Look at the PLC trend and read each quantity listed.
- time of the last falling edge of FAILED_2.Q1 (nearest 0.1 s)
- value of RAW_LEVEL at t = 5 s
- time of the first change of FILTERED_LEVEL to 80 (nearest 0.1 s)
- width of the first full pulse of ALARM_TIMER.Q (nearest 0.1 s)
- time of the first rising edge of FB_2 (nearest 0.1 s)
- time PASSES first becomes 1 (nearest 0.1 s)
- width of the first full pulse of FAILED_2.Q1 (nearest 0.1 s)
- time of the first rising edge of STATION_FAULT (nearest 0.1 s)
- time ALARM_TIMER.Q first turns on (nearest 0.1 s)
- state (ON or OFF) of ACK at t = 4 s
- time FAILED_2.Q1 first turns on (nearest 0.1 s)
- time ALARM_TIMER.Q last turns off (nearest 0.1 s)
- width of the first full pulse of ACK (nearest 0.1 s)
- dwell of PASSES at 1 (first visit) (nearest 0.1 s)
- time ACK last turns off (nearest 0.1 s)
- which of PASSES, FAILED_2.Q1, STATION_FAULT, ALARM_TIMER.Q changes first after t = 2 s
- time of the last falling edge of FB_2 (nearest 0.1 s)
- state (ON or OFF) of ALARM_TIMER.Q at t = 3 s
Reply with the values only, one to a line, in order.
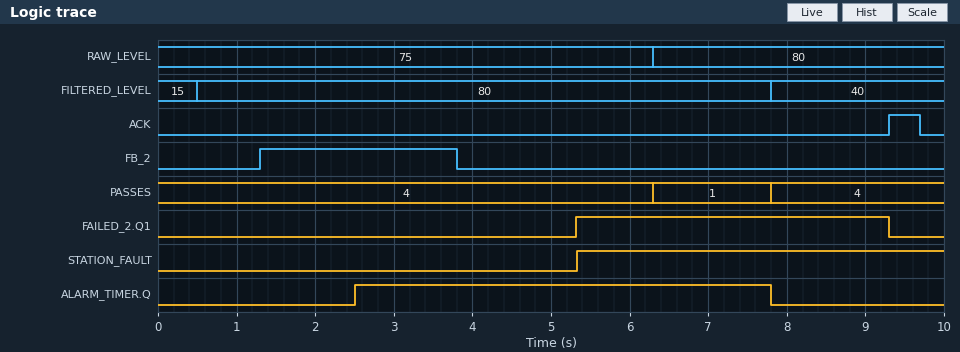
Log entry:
9.3 s
75
0.5 s
5.3 s
1.3 s
6.3 s
4.0 s
5.3 s
2.5 s
OFF
5.3 s
7.8 s
0.4 s
1.5 s
9.7 s
ALARM_TIMER.Q
3.8 s
ON
